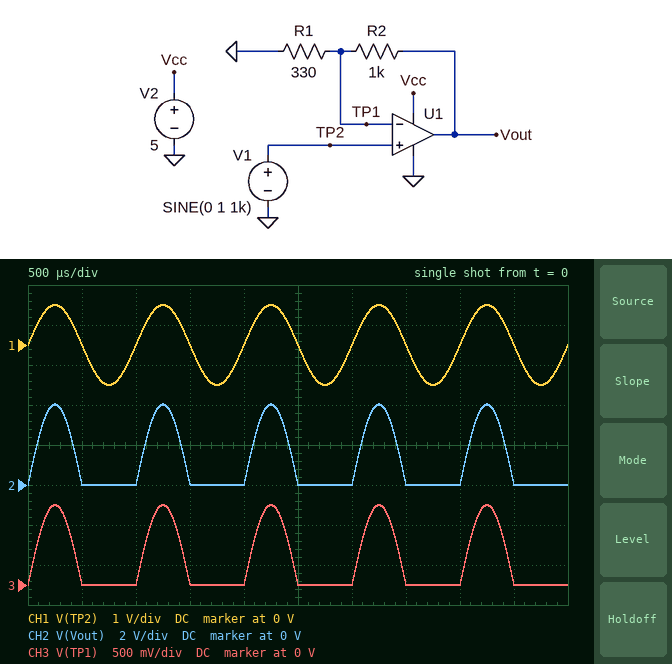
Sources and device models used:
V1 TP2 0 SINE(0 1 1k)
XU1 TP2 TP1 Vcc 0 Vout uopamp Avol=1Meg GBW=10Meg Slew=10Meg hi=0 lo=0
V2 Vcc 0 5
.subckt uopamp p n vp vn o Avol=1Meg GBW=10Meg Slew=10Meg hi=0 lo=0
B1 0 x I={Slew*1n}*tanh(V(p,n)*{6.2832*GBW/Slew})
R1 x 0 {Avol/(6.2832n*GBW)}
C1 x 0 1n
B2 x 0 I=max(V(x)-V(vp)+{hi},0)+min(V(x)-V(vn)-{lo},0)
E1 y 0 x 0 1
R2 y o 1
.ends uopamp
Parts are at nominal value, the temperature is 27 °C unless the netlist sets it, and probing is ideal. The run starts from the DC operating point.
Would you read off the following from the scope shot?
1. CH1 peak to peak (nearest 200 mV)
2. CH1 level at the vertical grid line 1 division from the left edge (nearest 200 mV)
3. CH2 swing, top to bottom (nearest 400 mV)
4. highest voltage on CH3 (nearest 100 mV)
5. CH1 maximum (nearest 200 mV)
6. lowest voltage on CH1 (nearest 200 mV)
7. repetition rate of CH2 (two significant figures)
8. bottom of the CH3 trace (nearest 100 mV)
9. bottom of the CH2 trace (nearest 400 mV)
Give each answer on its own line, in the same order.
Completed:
2.0 V
0 V
4.0 V
1.0 V
1.0 V
-1.0 V
1.0 kHz
0 V
0 V
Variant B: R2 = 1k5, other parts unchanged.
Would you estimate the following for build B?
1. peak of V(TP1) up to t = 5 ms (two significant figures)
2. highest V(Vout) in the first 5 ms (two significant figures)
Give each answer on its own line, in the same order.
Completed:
900 mV
5.0 V
